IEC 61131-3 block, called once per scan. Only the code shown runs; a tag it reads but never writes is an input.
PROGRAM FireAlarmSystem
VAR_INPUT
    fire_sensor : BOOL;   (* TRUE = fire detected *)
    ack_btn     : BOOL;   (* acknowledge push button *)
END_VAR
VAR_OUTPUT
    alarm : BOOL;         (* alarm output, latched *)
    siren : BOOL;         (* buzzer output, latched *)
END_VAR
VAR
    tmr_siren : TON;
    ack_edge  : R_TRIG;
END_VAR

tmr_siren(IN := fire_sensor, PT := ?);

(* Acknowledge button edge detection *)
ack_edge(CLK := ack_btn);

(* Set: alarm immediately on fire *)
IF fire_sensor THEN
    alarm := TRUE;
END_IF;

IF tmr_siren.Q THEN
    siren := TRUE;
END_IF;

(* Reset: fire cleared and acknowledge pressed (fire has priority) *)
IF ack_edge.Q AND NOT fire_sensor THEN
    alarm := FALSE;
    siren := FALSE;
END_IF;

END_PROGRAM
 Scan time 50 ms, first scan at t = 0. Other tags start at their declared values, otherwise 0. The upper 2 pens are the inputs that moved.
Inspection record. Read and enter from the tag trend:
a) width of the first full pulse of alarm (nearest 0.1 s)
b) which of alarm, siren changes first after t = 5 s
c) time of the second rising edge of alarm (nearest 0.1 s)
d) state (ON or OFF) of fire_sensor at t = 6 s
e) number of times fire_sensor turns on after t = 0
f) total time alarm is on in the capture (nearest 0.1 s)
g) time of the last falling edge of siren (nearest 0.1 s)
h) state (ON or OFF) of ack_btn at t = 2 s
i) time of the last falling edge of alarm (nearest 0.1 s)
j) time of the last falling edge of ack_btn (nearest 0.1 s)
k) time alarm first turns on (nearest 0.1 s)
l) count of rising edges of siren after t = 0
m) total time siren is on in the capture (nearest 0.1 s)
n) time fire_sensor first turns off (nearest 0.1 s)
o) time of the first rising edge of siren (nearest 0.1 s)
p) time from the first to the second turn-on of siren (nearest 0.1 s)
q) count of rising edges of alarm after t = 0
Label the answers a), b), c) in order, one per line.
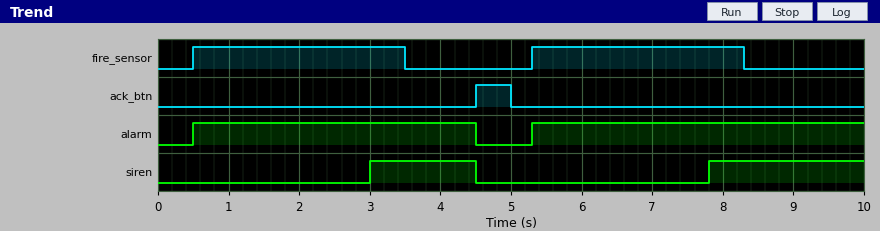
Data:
a) 4.0 s
b) alarm
c) 5.3 s
d) ON
e) 2
f) 8.7 s
g) 4.5 s
h) OFF
i) 4.5 s
j) 5.0 s
k) 0.5 s
l) 2
m) 3.7 s
n) 3.5 s
o) 3.0 s
p) 4.8 s
q) 2
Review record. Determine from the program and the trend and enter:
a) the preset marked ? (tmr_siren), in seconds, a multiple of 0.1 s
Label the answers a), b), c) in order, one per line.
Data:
a) 2.5 s
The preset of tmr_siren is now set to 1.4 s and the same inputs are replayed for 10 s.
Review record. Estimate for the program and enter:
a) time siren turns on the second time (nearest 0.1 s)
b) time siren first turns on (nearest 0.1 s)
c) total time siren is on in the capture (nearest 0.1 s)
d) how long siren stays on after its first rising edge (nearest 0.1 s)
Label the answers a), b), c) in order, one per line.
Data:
a) 6.7 s
b) 1.9 s
c) 5.9 s
d) 2.6 s
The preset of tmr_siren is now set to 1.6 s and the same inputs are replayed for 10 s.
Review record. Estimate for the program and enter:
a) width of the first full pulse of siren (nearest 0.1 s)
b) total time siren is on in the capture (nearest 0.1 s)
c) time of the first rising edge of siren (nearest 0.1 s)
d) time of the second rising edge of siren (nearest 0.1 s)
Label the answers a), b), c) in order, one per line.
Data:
a) 2.4 s
b) 5.5 s
c) 2.1 s
d) 6.9 s
